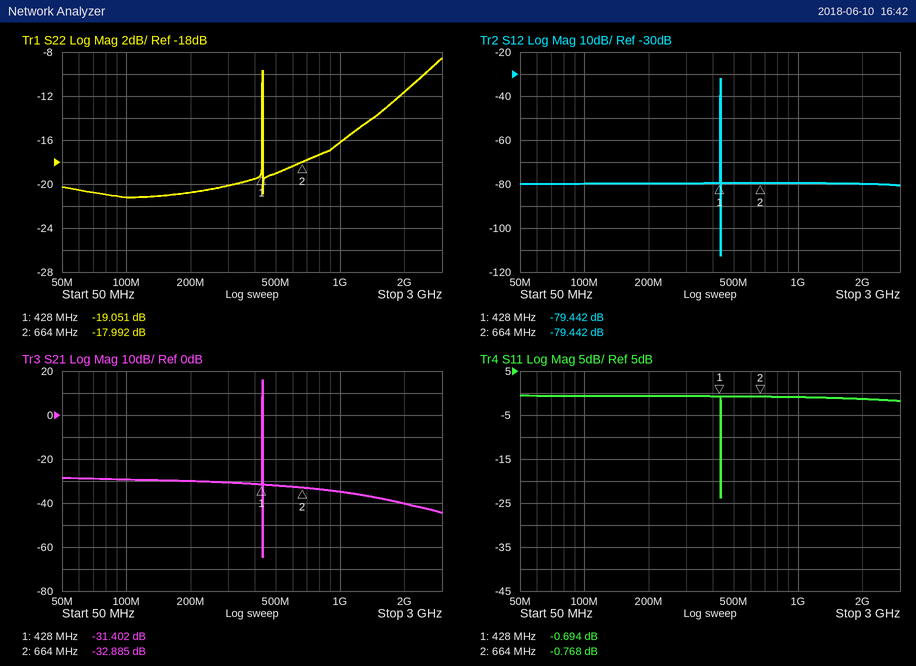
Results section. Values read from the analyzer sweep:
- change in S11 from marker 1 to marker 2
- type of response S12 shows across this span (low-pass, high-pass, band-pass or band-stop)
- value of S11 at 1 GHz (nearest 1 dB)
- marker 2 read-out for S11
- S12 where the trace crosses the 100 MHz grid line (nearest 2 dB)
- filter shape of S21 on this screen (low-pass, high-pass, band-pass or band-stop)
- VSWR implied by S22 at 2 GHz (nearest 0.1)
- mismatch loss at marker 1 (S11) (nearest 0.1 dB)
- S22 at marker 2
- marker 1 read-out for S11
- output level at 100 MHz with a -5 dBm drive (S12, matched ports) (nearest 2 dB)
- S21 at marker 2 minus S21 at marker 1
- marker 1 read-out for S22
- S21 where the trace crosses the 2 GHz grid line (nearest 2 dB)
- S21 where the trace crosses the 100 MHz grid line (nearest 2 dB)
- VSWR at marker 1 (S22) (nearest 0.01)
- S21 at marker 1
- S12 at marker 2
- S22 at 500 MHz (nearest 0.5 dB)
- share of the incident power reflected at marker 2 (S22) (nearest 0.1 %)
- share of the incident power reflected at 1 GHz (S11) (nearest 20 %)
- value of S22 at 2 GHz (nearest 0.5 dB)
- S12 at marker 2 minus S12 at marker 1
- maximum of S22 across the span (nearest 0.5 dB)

-0.074 dB
band-pass
-1 dB
-0.768 dB
-80 dB
band-pass
1.7
8.3 dB
-17.992 dB
-0.694 dB
-84 dBm
-1.483 dB
-19.051 dB
-40 dB
-30 dB
1.25
-31.402 dB
-79.442 dB
-19.0 dB
1.6 %
80 %
-11.5 dB
0.000 dB
-8.5 dB
